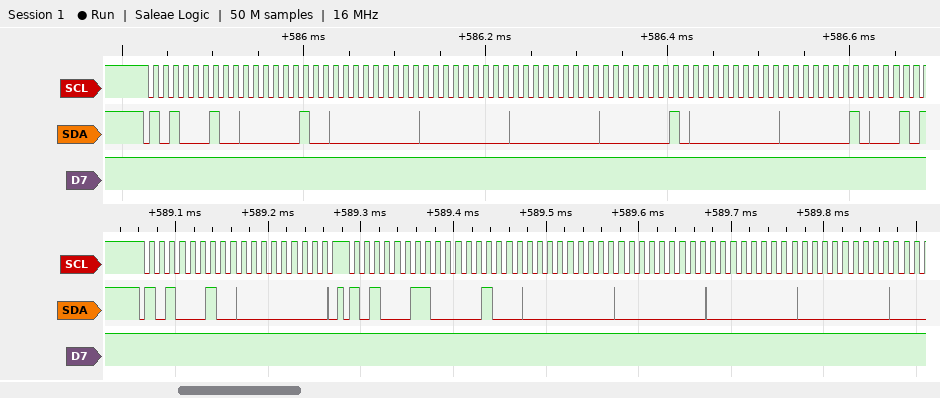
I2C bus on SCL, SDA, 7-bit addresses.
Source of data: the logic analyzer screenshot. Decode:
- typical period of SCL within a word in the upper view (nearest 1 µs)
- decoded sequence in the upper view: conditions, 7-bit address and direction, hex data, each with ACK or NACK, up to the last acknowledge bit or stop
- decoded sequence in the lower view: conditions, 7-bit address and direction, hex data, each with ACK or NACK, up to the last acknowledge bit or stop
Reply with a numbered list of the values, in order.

1. 11 µs
2. start, address 51 write ACK, 02 ACK, 00 ACK, 00 ACK, 00 ACK, 01 ACK, 00 ACK, 01 ACK
3. start, address 51 write ACK, 00 ACK, stop, start, address 51 read ACK, 08 ACK, 00 ACK, 00 ACK, 00 ACK, 00 ACK
